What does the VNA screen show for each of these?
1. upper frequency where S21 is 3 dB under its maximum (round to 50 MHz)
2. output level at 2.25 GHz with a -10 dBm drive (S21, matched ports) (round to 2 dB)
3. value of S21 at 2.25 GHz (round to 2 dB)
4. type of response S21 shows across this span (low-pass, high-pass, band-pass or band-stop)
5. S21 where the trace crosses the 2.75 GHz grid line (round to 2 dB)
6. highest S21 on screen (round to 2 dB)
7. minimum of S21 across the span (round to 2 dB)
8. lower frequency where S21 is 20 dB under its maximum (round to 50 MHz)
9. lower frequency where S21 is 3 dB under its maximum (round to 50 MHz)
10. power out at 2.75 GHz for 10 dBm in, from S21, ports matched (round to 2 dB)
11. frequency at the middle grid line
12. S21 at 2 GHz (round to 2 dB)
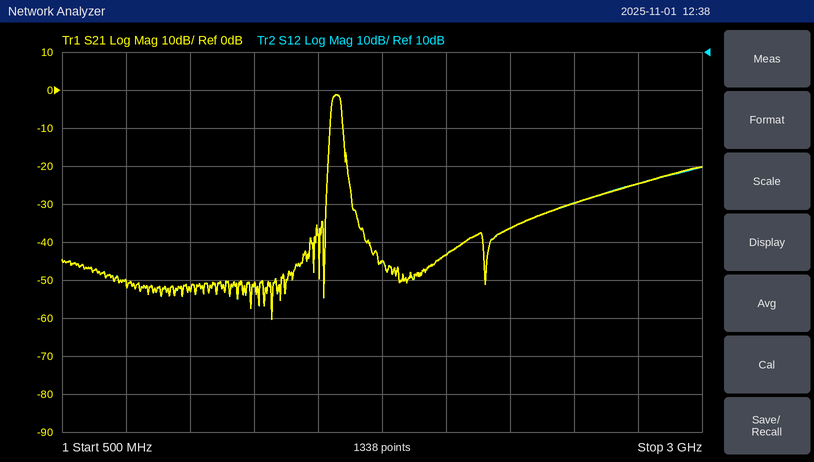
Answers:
1.60 GHz
-46 dBm
-36 dB
band-pass
-24 dB
-2 dB
-60 dB
1.55 GHz
1.55 GHz
-14 dBm
1.75 GHz
-44 dB
